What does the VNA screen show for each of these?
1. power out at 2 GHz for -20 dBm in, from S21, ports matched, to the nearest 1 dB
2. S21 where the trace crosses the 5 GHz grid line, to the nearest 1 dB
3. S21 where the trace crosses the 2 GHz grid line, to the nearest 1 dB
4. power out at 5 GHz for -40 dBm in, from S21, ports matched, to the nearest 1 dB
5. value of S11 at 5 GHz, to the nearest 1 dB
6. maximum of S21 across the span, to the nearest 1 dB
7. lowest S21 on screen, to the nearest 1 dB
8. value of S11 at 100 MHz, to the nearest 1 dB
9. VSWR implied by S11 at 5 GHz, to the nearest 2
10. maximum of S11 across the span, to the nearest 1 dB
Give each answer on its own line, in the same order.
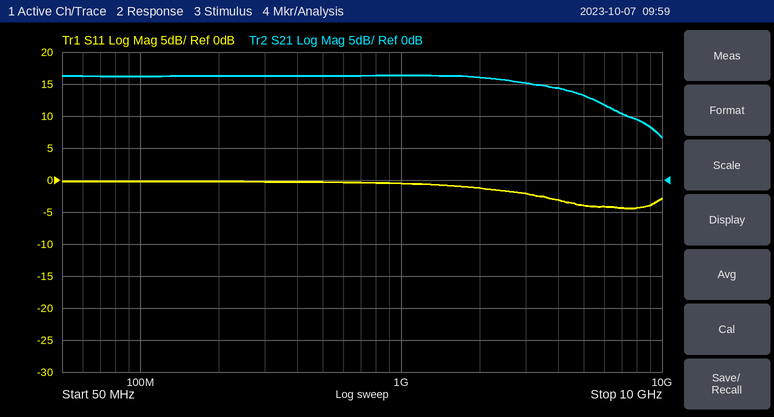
-4 dBm
13 dB
16 dB
-27 dBm
-4 dB
16 dB
7 dB
0 dB
4
0 dB
